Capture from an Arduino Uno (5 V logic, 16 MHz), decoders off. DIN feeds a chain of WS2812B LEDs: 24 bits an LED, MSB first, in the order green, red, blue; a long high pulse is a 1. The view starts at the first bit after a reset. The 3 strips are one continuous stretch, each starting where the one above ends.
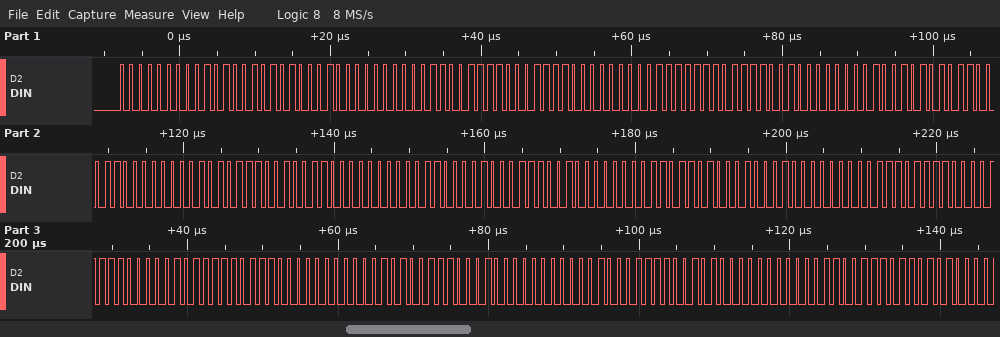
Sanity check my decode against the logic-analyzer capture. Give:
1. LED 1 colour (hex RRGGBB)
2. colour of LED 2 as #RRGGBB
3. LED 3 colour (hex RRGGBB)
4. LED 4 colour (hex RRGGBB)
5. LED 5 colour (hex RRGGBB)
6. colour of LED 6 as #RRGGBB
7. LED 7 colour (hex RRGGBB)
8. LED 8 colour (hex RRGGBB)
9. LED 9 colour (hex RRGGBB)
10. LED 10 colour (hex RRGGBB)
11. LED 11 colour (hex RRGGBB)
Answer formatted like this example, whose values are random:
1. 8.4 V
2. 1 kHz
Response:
1. #5200A2
2. #67008F
3. #7F0079
4. #950063
5. #AE004C
6. #C20039
7. #DA0022
8. #EF000F
9. #F70500
10. #E21400
11. #CA2300
